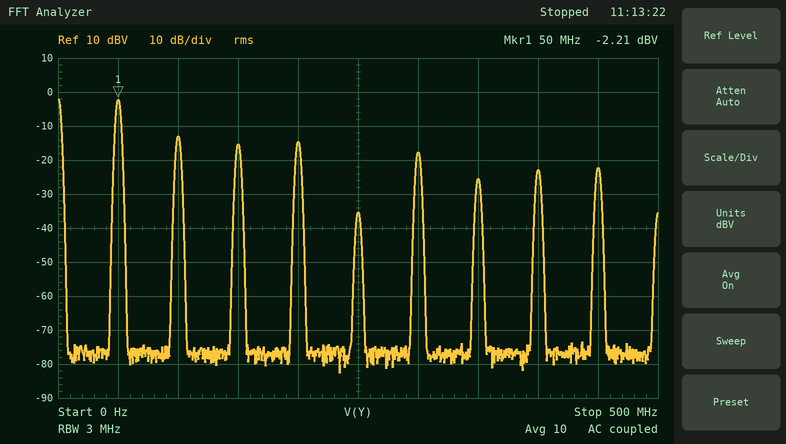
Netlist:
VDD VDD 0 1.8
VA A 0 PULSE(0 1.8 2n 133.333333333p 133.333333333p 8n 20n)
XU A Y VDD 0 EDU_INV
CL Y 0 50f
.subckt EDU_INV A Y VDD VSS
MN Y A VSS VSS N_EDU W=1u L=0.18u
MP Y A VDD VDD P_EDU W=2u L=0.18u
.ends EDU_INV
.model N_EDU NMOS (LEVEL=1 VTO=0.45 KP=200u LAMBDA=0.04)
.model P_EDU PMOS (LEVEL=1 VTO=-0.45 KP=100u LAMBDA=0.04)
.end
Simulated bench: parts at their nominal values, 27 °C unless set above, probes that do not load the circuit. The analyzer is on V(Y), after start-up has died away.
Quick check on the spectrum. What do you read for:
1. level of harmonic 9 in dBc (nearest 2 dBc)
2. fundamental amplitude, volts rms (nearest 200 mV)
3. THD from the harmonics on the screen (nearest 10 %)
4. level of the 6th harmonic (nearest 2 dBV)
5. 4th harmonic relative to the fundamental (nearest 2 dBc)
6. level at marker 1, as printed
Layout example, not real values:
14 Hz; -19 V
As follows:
-20 dBc; 800 mV; 50 %; -18 dBV; -12 dBc; -2.21 dBV
